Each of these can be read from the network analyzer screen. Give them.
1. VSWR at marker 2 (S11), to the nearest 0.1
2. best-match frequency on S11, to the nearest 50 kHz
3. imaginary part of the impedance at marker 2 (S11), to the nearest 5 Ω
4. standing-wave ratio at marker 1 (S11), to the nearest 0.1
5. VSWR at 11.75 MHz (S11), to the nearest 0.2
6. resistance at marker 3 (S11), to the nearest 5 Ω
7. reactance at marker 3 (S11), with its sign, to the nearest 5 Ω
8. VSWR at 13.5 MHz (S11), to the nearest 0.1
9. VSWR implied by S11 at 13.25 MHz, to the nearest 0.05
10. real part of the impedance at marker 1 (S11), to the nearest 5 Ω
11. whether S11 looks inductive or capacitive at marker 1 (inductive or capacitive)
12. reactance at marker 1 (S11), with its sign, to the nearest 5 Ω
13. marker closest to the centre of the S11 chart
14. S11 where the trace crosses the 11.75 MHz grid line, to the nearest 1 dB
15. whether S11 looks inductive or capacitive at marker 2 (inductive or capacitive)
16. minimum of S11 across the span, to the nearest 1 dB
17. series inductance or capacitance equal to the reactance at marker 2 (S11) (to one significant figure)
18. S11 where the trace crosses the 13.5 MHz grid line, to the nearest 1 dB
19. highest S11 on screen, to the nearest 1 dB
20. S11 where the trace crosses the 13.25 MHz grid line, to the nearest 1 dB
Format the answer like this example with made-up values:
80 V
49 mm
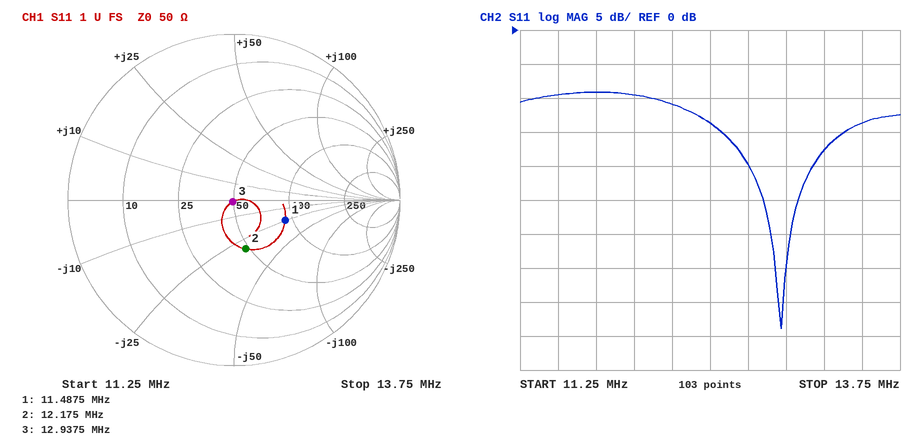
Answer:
1.9
12.95 MHz
-30 Ω
2.0
2.0
50 Ω
0 Ω
1.5
1.30
90 Ω
capacitive
-25 Ω
marker 3
-9 dB
capacitive
-44 dB
400 pF
-14 dB
-9 dB
-18 dB
